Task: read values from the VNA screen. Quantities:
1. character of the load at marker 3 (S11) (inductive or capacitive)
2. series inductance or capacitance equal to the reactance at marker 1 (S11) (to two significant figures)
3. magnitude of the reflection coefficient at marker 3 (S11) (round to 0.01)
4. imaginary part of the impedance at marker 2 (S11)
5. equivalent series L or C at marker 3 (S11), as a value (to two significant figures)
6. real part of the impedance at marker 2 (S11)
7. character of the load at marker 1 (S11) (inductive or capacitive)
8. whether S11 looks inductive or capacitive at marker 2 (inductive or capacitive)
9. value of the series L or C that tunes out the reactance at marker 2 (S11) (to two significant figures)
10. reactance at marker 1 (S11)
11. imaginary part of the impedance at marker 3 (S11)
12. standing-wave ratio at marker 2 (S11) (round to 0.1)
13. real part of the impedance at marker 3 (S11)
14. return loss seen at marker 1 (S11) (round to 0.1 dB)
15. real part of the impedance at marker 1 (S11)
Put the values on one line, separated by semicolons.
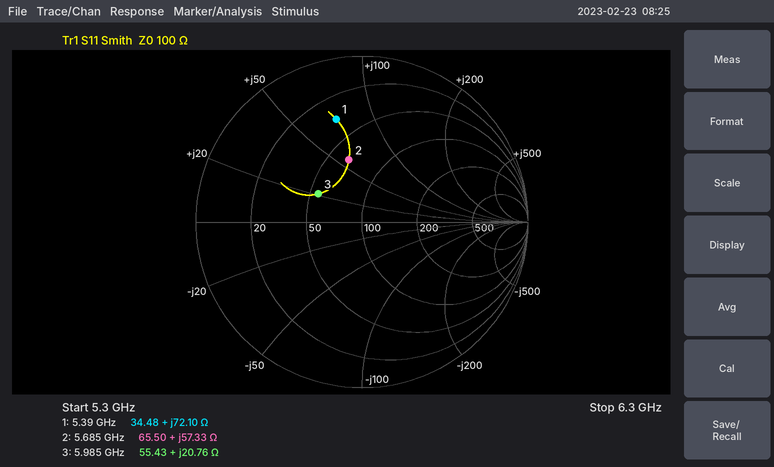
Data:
inductive; 2.1 nH; 0.31; +57.33 Ω; 550 pH; 65.50 Ω; inductive; inductive; 490 fF; +72.10 Ω; +20.76 Ω; 2.2; 55.43 Ω; 3.9 dB; 34.48 Ω
